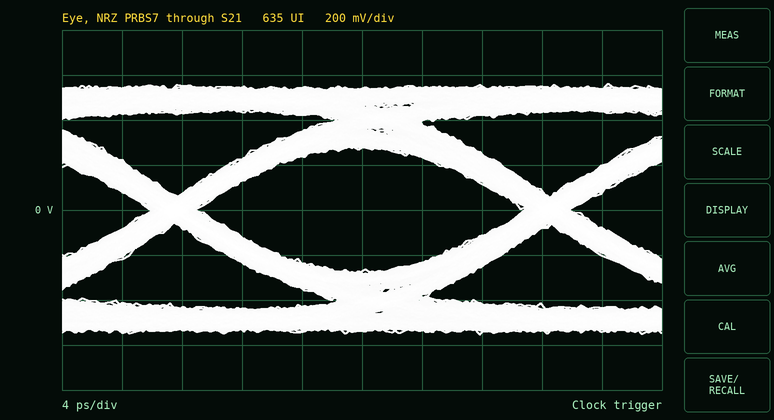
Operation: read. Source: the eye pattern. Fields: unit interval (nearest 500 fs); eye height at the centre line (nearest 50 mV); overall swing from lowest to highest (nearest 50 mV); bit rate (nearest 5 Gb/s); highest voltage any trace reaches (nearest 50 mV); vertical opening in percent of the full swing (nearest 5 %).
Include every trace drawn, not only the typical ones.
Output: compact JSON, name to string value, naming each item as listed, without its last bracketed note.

{"unit interval": "25.0 ps", "eye height at the centre line": "550 mV", "overall swing from lowest to highest": "1.10 V", "bit rate": "40 Gb/s", "highest voltage any trace reaches": "550 mV", "vertical opening in percent of the full swing": "50 %"}
